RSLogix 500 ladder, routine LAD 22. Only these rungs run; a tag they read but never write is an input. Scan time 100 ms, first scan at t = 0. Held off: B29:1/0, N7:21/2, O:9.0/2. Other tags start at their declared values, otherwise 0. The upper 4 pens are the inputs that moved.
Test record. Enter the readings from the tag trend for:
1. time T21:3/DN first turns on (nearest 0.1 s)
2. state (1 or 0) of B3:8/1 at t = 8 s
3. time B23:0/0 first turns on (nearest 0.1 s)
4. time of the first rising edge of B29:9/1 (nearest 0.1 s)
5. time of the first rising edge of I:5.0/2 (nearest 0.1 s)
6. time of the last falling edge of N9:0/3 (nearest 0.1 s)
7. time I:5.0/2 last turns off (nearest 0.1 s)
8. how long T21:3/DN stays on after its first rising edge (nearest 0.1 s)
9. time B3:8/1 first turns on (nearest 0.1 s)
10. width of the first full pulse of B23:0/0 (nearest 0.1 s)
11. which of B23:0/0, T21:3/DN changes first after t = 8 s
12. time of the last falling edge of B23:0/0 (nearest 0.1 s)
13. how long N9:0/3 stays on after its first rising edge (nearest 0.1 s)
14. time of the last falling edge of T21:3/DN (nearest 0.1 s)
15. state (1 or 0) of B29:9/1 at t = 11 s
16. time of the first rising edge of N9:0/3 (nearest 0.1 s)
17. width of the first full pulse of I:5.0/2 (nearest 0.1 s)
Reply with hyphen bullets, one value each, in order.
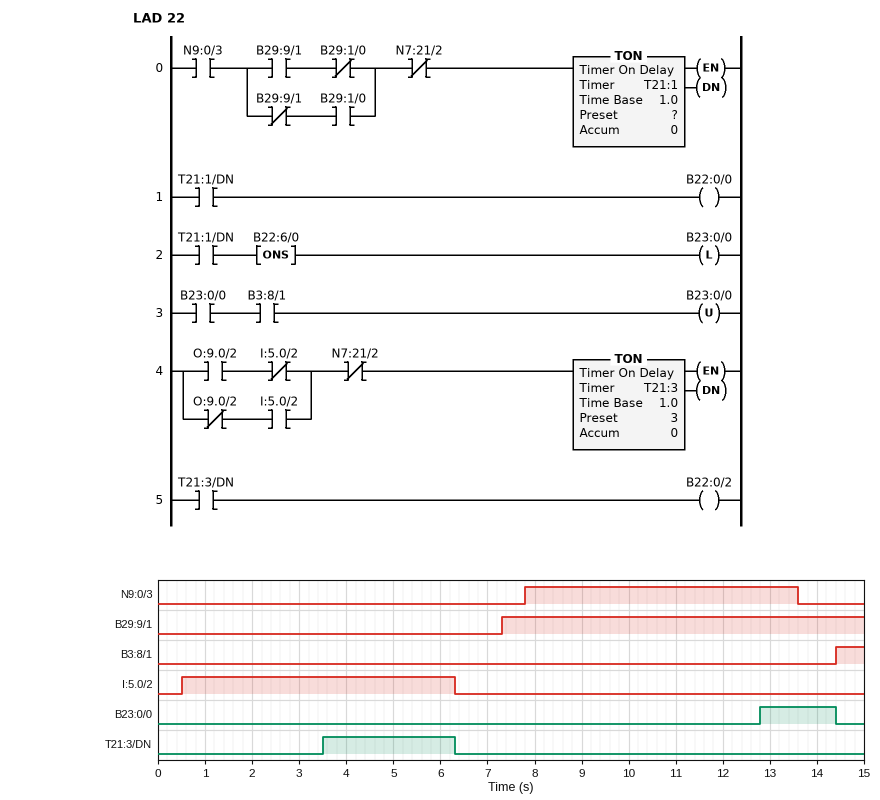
- 3.5 s
- 0
- 12.8 s
- 7.3 s
- 0.5 s
- 13.6 s
- 6.3 s
- 2.8 s
- 14.4 s
- 1.6 s
- B23:0/0
- 14.4 s
- 5.8 s
- 6.3 s
- 1
- 7.8 s
- 5.8 s
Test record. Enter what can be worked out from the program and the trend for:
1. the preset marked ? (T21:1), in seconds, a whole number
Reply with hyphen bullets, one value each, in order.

- 5 s
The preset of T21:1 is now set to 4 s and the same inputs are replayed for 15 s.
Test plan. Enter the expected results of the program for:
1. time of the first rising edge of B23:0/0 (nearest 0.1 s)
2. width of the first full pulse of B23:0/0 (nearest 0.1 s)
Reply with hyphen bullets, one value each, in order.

- 11.8 s
- 2.6 s
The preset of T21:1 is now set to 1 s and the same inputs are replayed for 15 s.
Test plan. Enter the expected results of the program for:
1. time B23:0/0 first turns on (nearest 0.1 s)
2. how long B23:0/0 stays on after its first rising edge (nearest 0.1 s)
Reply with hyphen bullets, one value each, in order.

- 8.8 s
- 5.6 s
